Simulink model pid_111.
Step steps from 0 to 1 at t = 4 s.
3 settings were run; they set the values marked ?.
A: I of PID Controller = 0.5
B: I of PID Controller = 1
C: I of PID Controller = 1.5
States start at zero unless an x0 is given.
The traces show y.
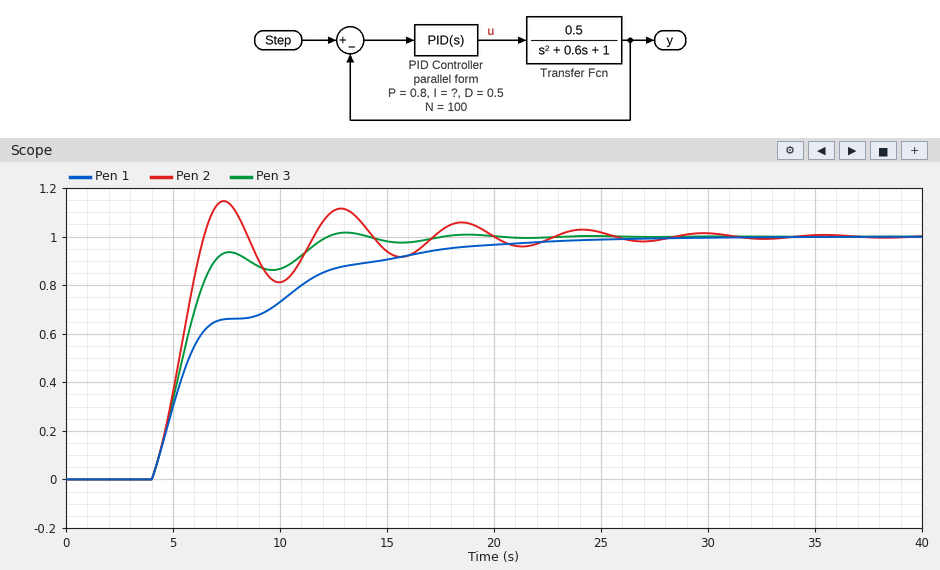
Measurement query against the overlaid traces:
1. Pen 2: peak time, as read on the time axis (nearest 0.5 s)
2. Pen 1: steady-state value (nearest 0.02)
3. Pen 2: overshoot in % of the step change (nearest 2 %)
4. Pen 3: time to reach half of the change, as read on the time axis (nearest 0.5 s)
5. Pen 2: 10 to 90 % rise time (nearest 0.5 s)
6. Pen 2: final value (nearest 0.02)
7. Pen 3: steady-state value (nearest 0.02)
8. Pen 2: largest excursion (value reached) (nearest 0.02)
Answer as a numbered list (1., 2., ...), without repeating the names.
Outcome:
1. 7.5 s
2. 1.00
3. 14 %
4. 5.5 s
5. 2.0 s
6. 1.00
7. 1.00
8. 1.14
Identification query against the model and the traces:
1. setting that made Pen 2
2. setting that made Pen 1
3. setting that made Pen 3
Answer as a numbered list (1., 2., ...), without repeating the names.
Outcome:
1. C
2. A
3. B
